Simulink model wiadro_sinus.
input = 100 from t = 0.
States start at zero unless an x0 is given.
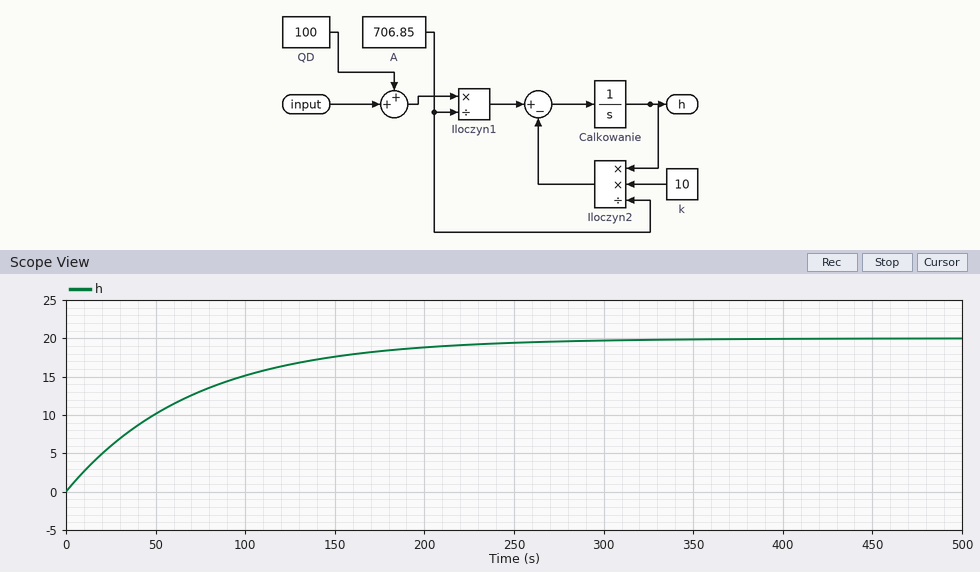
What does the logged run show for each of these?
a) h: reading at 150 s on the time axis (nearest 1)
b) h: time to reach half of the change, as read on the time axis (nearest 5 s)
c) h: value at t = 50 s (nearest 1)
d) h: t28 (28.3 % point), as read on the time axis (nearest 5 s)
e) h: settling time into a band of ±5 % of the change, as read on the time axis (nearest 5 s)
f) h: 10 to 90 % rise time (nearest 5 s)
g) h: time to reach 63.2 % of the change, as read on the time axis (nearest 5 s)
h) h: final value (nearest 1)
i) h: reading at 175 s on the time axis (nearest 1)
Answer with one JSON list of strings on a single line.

["18", "50 s", "10", "25 s", "210 s", "155 s", "70 s", "20", "18"]
